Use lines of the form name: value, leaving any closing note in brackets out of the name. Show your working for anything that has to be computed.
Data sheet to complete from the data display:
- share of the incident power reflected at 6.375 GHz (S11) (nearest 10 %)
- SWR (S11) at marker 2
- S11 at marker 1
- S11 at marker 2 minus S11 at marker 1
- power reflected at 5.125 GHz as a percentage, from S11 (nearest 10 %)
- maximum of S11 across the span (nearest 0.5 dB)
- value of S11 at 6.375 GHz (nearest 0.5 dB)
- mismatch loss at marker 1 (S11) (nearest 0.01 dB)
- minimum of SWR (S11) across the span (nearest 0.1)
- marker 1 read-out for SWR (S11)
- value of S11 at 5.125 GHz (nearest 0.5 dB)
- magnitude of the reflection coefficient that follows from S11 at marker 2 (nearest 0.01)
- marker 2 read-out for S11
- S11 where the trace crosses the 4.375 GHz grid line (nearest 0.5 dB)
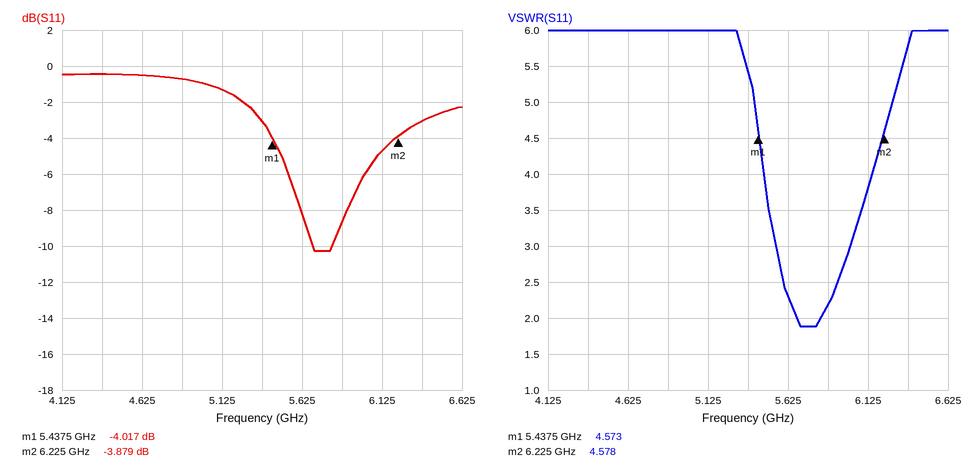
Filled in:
share of the incident power reflected at 6.375 GHz (S11): 10^(-3/10) ≈ 50 %
SWR (S11) at marker 2: 4.578
S11 at marker 1: -4.017 dB
S11 at marker 2 minus S11 at marker 1: -3.879 − (-4.017) = 0.138 dB
power reflected at 5.125 GHz as a percentage, from S11: 10^(-1.5/10) ≈ 70.8 %, so 70 % to the nearest 10 %
maximum of S11 across the span: -0.5 dB
value of S11 at 6.375 GHz: -3.0 dB
mismatch loss at marker 1 (S11): −10 log10(1 − 10^(-4.017/10)) ≈ 2.19 dB
minimum of SWR (S11) across the span: 1.9
marker 1 read-out for SWR: 4.573
value of S11 at 5.125 GHz: -1.5 dB
magnitude of the reflection coefficient that follows from S11 at marker 2: 10^(-3.879/20) ≈ 0.64
marker 2 read-out for S11: -3.879 dB
S11 where the trace crosses the 4.375 GHz grid line: -0.5 dB
